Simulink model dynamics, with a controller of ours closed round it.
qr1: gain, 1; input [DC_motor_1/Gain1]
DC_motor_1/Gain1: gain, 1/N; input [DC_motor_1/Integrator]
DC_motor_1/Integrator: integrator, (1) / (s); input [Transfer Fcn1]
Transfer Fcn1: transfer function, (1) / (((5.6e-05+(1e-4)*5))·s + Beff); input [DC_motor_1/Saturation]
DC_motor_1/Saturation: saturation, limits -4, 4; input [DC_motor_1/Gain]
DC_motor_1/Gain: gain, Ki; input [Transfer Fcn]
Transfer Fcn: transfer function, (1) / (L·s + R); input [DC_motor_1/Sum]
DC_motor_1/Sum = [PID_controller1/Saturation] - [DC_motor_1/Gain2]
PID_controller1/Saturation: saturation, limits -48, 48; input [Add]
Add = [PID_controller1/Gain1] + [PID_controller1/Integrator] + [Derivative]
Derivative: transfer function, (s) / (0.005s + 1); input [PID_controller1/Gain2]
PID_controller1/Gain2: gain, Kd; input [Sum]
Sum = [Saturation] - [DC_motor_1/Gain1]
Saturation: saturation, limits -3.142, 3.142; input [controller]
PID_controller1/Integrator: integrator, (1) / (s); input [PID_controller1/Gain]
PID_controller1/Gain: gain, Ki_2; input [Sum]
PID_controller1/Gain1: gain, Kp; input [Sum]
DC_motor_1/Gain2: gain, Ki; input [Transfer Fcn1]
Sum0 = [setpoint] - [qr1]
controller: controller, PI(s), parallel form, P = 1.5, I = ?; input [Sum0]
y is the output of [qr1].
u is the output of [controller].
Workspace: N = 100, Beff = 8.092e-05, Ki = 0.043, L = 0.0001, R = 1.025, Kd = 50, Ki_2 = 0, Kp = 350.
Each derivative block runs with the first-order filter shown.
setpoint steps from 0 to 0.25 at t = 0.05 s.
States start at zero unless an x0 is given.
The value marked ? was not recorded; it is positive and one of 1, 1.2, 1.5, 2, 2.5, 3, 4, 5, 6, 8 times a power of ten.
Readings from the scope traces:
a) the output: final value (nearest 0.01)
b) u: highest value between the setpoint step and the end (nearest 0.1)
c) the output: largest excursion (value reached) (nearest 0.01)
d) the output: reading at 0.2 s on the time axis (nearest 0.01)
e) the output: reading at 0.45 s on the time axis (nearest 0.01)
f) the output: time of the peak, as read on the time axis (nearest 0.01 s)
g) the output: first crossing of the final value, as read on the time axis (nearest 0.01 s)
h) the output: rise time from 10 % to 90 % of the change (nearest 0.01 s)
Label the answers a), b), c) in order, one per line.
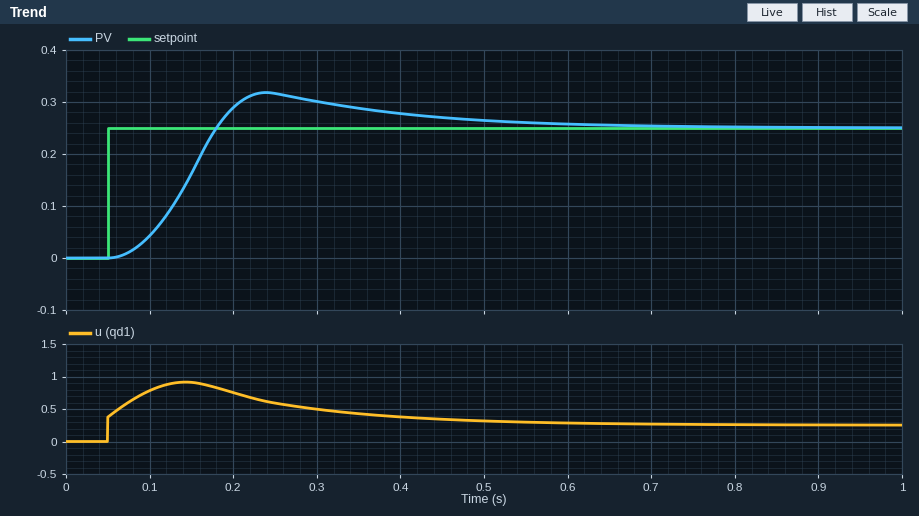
a) 0.25
b) 0.9
c) 0.32
d) 0.29
e) 0.27
f) 0.24 s
g) 0.18 s
h) 0.08 s
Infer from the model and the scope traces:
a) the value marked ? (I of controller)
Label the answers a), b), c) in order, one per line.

a) 40
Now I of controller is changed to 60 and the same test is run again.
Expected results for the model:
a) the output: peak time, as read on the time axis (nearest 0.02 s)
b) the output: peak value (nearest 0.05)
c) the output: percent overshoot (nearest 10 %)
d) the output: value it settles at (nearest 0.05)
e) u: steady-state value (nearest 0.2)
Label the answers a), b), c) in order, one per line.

a) 0.26 s
b) 0.40
c) 60 %
d) 0.25
e) 0.2
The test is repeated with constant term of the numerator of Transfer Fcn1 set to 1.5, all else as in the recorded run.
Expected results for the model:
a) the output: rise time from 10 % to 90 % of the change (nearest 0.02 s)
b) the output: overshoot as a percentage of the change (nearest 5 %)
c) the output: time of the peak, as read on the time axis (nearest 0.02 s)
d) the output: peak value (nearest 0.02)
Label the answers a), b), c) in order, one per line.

a) 0.08 s
b) 15 %
c) 0.26 s
d) 0.30
